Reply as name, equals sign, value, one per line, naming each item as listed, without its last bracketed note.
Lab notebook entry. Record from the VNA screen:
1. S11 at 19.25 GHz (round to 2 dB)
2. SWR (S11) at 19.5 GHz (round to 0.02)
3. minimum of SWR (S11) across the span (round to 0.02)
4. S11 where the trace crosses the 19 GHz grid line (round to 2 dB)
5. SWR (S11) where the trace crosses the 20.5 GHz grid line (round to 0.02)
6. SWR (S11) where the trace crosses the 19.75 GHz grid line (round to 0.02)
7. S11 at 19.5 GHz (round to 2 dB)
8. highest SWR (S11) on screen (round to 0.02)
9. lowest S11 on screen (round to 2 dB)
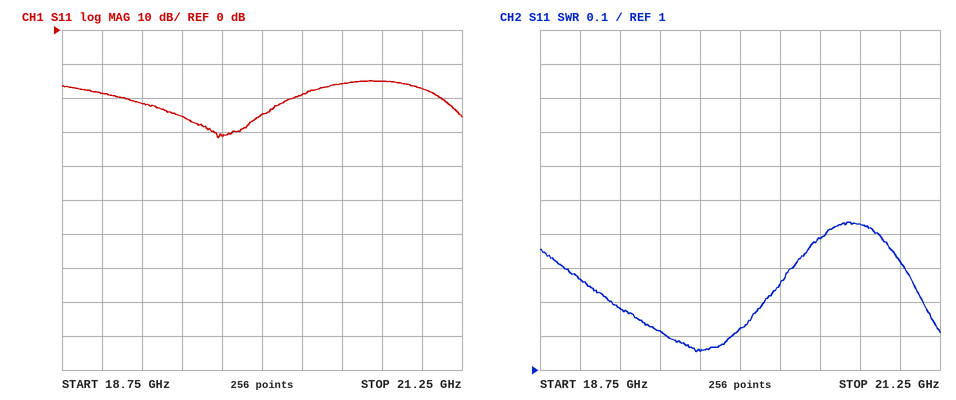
S11 at 19.25 GHz = -22 dB
SWR (S11) at 19.5 GHz = 1.12
minimum of SWR (S11) across the span = 1.06
S11 where the trace crosses the 19 GHz grid line = -18 dB
SWR (S11) where the trace crosses the 20.5 GHz grid line = 1.38
SWR (S11) where the trace crosses the 19.75 GHz grid line = 1.06
S11 at 19.5 GHz = -26 dB
highest SWR (S11) on screen = 1.44
lowest S11 on screen = -32 dB
